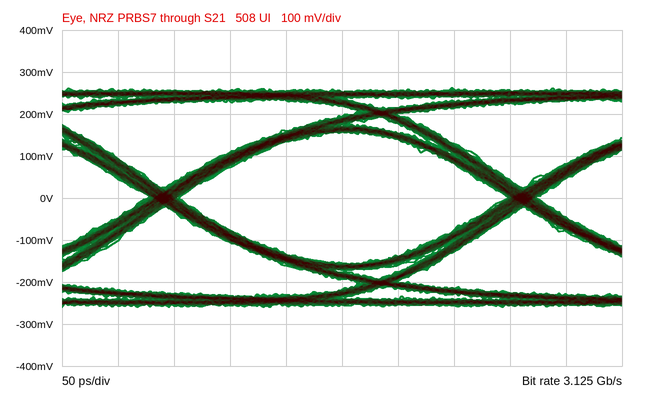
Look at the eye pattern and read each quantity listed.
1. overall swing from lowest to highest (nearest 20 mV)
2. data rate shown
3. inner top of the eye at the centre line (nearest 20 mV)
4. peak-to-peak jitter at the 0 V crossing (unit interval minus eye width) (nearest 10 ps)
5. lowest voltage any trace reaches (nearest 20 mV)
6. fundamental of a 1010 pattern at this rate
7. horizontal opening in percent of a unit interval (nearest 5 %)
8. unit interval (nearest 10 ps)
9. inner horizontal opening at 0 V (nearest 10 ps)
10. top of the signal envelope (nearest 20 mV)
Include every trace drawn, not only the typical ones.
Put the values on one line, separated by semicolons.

520 mV; 3.125 Gb/s; 160 mV; 30 ps; -260 mV; 1.5625 GHz; 90 %; 320 ps; 290 ps; 260 mV
